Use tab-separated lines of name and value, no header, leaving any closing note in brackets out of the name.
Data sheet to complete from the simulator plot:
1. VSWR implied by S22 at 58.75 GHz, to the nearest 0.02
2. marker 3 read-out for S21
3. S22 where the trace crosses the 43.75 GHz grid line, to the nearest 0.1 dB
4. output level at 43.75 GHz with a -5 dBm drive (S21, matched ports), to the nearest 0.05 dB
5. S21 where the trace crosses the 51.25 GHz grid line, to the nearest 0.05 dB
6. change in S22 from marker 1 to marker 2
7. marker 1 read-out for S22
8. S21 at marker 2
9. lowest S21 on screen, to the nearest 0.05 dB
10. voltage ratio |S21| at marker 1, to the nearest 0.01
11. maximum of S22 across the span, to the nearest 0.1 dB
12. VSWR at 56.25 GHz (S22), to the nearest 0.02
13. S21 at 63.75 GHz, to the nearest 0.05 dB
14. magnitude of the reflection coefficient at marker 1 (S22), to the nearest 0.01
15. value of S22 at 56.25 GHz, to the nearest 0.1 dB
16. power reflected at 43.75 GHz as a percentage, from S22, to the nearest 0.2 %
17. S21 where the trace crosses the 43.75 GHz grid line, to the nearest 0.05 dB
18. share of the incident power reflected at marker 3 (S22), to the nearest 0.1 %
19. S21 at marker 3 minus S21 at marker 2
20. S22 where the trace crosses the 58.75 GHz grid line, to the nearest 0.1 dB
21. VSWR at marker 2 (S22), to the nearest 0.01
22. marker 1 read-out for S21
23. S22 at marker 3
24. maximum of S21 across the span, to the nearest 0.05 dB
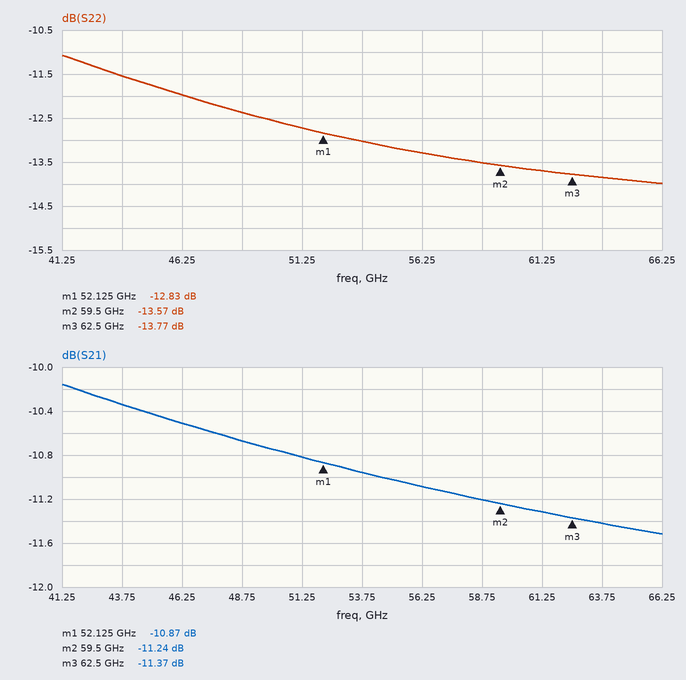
VSWR implied by S22 at 58.75 GHz, to the nearest 0.02	1.54
marker 3 read-out for S21	-11.37 dB
S22 where the trace crosses the 43.75 GHz grid line, to the nearest 0.1 dB	-11.5 dB
output level at 43.75 GHz with a -5 dBm drive (S21, matched ports), to the nearest 0.05 dB	-15.35 dBm
S21 where the trace crosses the 51.25 GHz grid line, to the nearest 0.05 dB	-10.80 dB
change in S22 from marker 1 to marker 2	-0.74 dB
marker 1 read-out for S22	-12.83 dB
S21 at marker 2	-11.24 dB
lowest S21 on screen, to the nearest 0.05 dB	-11.50 dB
voltage ratio |S21| at marker 1, to the nearest 0.01	0.29
maximum of S22 across the span, to the nearest 0.1 dB	-11.1 dB
VSWR at 56.25 GHz (S22), to the nearest 0.02	1.56
S21 at 63.75 GHz, to the nearest 0.05 dB	-11.40 dB
magnitude of the reflection coefficient at marker 1 (S22), to the nearest 0.01	0.23
value of S22 at 56.25 GHz, to the nearest 0.1 dB	-13.3 dB
power reflected at 43.75 GHz as a percentage, from S22, to the nearest 0.2 %	7.0 %
S21 where the trace crosses the 43.75 GHz grid line, to the nearest 0.05 dB	-10.35 dB
share of the incident power reflected at marker 3 (S22), to the nearest 0.1 %	4.2 %
S21 at marker 3 minus S21 at marker 2	-0.13 dB
S22 where the trace crosses the 58.75 GHz grid line, to the nearest 0.1 dB	-13.5 dB
VSWR at marker 2 (S22), to the nearest 0.01	1.53
marker 1 read-out for S21	-10.87 dB
S22 at marker 3	-13.77 dB
maximum of S21 across the span, to the nearest 0.05 dB	-10.15 dB
